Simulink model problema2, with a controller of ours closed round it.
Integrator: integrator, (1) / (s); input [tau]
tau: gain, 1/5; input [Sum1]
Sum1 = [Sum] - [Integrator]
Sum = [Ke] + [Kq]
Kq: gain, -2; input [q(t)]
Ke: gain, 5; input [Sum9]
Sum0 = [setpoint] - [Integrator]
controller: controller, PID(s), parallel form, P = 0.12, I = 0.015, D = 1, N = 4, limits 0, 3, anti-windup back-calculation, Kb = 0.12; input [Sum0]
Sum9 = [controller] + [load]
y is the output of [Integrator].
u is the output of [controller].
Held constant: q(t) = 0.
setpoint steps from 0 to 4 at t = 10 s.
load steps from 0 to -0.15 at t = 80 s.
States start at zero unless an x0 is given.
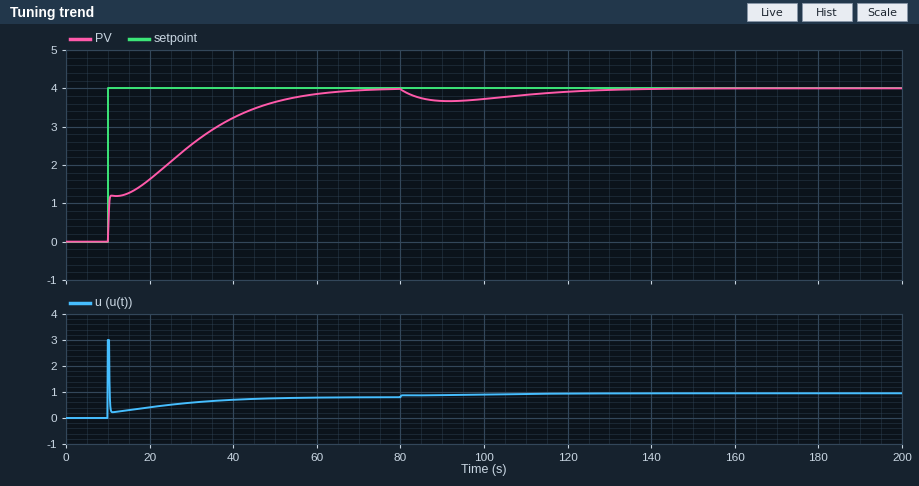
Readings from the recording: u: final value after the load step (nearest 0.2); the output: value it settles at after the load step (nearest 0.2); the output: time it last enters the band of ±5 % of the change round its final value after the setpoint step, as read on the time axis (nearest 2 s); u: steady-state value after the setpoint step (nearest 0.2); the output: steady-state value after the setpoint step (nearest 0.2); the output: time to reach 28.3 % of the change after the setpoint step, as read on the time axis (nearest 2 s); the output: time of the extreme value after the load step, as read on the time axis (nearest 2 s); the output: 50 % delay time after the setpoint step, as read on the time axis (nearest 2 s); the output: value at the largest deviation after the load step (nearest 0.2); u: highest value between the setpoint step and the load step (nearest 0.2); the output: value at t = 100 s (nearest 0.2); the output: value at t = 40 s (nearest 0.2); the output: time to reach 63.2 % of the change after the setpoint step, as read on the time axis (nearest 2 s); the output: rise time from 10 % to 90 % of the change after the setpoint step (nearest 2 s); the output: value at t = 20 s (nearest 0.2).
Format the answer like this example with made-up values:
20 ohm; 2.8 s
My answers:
1.0; 4.0; 56 s; 0.8; 4.0; 10 s; 92 s; 24 s; 3.6; 3.0; 3.8; 3.2; 30 s; 38 s; 1.6
